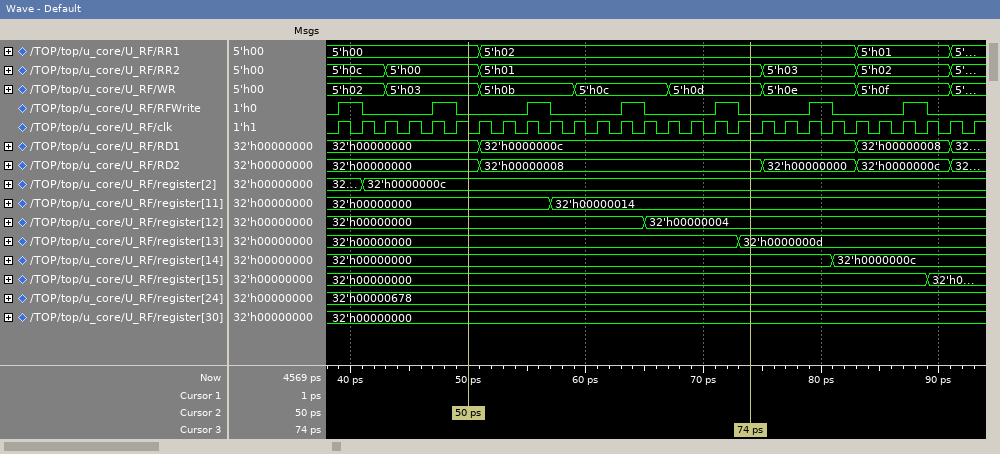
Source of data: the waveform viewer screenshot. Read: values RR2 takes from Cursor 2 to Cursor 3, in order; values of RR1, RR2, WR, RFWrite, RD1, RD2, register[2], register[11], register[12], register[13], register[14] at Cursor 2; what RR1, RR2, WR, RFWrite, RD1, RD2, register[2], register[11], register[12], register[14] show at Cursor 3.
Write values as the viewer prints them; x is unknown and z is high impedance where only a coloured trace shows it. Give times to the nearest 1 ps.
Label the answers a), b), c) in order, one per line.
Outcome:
a) 5'h00, 5'h01
b) RR1=5'h00, RR2=5'h00, WR=5'h03, RFWrite=0, RD1=32'h00000000, RD2=32'h00000000, register[2]=32'h0000000c, register[11]=32'h00000000, register[12]=32'h00000000, register[13]=32'h00000000, register[14]=32'h00000000
c) RR1=5'h02, RR2=5'h01, WR=5'h0d, RFWrite=0, RD1=32'h0000000c, RD2=32'h00000008, register[2]=32'h0000000c, register[11]=32'h00000014, register[12]=32'h00000004, register[14]=32'h00000000
